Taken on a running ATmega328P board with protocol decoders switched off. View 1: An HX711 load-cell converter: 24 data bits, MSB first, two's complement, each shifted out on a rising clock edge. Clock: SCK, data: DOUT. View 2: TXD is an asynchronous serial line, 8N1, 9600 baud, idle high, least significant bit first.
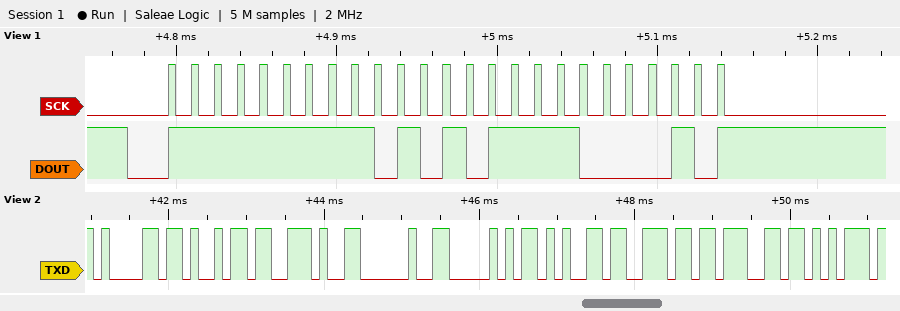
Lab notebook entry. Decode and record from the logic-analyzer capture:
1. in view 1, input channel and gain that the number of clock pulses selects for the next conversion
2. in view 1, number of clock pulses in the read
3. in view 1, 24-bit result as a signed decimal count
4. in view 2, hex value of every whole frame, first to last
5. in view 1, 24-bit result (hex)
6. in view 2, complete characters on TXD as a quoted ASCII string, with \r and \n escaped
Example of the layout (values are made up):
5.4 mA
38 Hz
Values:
channel A, gain 128
25
-21566
0x61 0x69 0x2E 0x20 0x50 0x65 0x6E 0x67 0x75
0xFFABC2
"ai. Pengu"
